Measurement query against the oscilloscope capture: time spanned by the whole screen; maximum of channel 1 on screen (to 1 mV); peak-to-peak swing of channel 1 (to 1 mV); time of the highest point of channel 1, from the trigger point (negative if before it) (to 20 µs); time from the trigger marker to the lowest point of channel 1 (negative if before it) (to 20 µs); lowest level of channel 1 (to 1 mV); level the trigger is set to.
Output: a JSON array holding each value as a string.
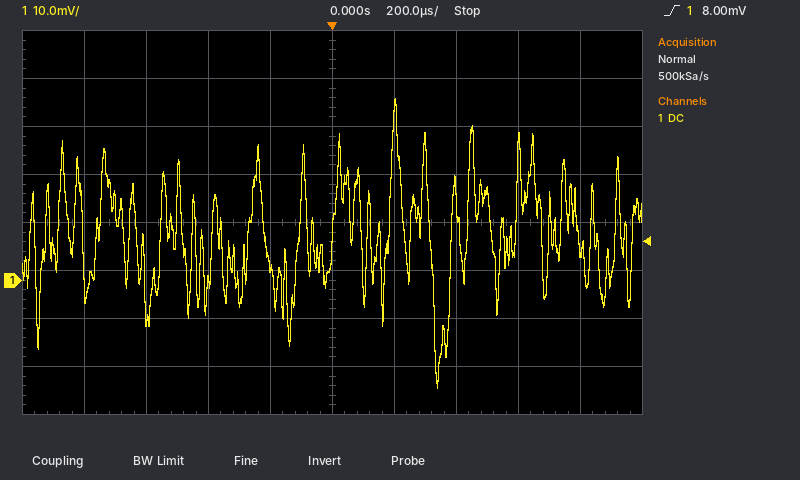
["2 ms", "38 mV", "60 mV", "+200 µs", "+340 µs", "-22 mV", "8.00 mV"]
